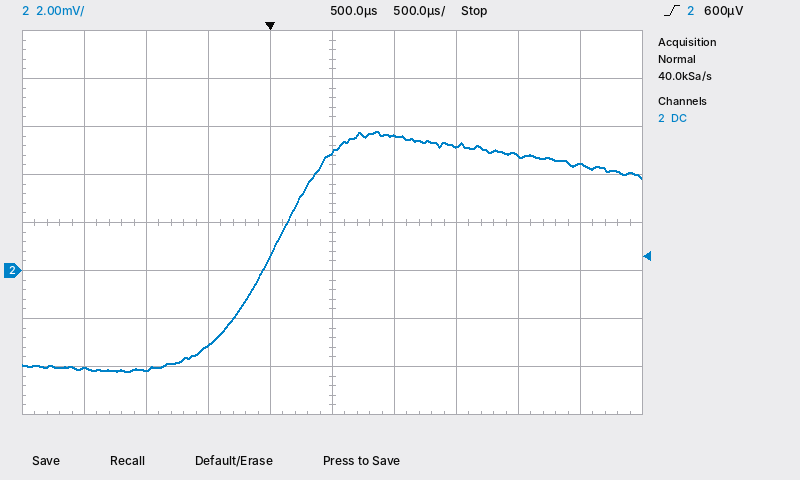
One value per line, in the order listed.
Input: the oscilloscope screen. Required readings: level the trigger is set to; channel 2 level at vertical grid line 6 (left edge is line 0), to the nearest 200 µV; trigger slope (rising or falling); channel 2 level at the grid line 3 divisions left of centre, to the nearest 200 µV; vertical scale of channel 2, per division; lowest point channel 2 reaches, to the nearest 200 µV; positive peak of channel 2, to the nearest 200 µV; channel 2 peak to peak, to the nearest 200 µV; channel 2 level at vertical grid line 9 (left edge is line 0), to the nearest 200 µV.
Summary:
600 µV
5.6 mV
rising
-4.2 mV
2 mV
-4.2 mV
5.8 mV
10.0 mV
4.4 mV
